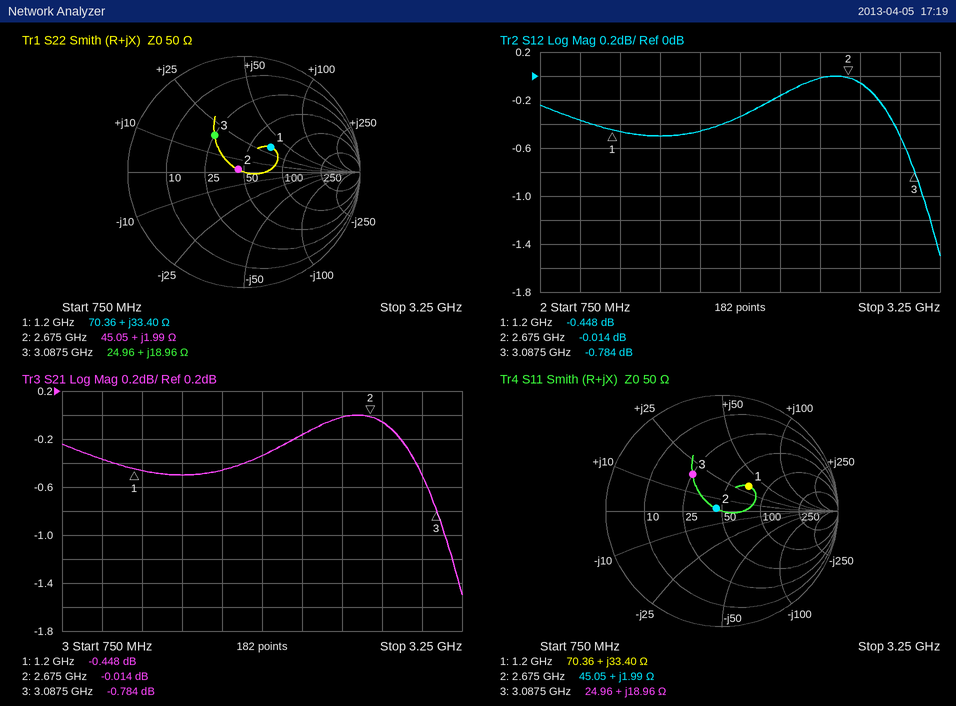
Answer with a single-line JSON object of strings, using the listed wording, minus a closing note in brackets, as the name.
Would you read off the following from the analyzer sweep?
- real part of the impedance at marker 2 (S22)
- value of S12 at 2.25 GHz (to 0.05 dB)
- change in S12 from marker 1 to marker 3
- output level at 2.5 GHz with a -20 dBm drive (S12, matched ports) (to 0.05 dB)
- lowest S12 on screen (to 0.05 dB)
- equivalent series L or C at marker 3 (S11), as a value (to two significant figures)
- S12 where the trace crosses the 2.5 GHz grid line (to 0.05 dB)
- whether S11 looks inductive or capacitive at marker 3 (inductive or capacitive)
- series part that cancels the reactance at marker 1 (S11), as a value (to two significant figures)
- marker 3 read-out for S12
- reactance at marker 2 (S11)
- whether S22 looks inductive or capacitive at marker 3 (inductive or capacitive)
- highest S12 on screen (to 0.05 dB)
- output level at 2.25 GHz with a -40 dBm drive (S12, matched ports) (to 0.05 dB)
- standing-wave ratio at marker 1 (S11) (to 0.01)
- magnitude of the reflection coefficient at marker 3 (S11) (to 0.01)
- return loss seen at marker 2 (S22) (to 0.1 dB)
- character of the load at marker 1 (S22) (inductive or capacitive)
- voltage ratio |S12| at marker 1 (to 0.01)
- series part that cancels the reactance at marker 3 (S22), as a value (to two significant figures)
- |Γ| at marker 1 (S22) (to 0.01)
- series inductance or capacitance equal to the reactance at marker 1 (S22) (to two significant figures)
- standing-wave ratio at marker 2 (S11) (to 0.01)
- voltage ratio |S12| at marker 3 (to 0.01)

{"real part of the impedance at marker 2": "45.05 Ω", "value of S12 at 2.25 GHz": "-0.15 dB", "change in S12 from marker 1 to marker 3": "-0.336 dB", "output level at 2.5 GHz with a -20 dBm drive (S12, matched ports)": "-20.00 dBm", "lowest S12 on screen": "-1.50 dB", "equivalent series L or C at marker 3 (S11), as a value": "980 pH", "S12 where the trace crosses the 2.5 GHz grid line": "0.00 dB", "whether S11 looks inductive or capacitive at marker 3": "inductive", "series part that cancels the reactance at marker 1 (S11), as a value": "4.0 pF", "marker 3 read-out for S12": "-0.784 dB", "reactance at marker 2": "+1.99 Ω", "whether S22 looks inductive or capacitive at marker 3": "inductive", "highest S12 on screen": "0.00 dB", "output level at 2.25 GHz with a -40 dBm drive (S12, matched ports)": "-40.15 dBm", "standing-wave ratio at marker 1 (S11)": "1.91", "magnitude of the reflection coefficient at marker 3 (S11)": "0.41", "return loss seen at marker 2 (S22)": "25.0 dB", "character of the load at marker 1 (S22)": "inductive", "voltage ratio |S12| at marker 1": "0.95", "series part that cancels the reactance at marker 3 (S22), as a value": "2.7 pF", "|Γ| at marker 1 (S22)": "0.31", "series inductance or capacitance equal to the reactance at marker 1 (S22)": "4.4 nH", "standing-wave ratio at marker 2 (S11)": "1.12", "voltage ratio |S12| at marker 3": "0.91"}
